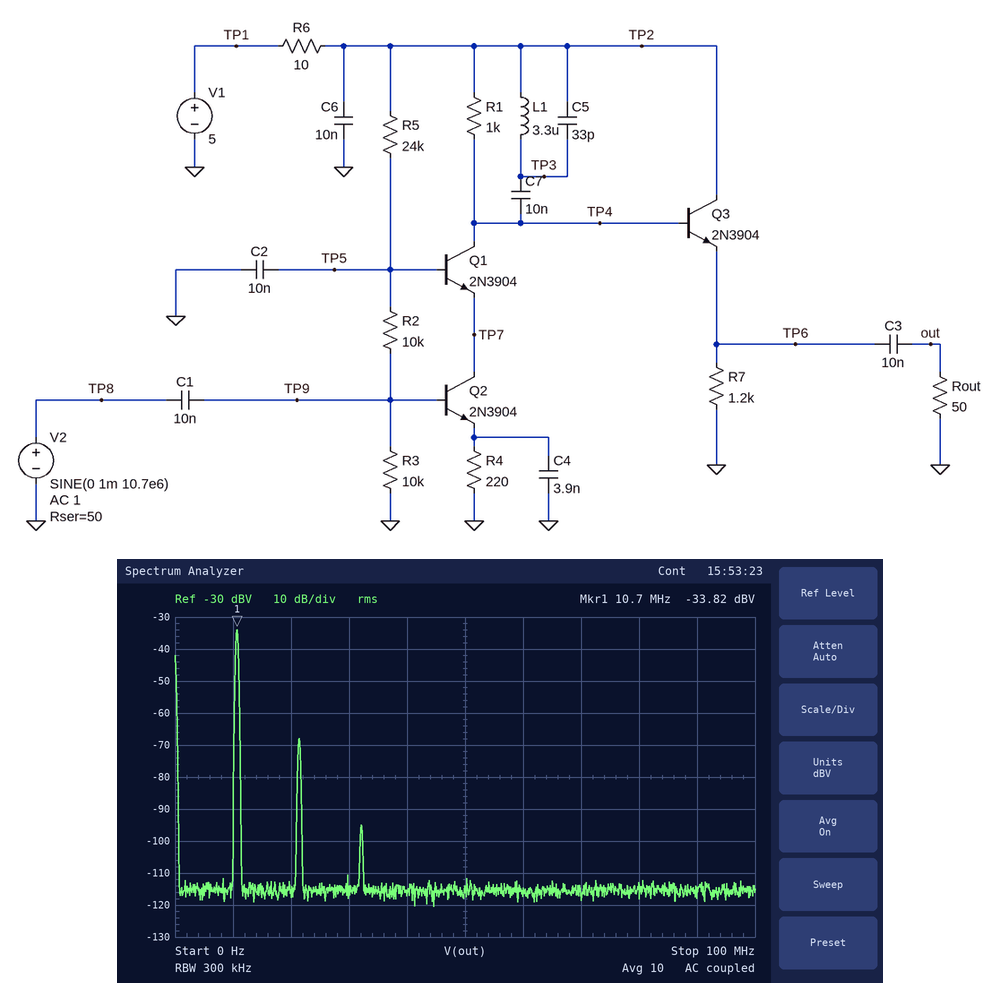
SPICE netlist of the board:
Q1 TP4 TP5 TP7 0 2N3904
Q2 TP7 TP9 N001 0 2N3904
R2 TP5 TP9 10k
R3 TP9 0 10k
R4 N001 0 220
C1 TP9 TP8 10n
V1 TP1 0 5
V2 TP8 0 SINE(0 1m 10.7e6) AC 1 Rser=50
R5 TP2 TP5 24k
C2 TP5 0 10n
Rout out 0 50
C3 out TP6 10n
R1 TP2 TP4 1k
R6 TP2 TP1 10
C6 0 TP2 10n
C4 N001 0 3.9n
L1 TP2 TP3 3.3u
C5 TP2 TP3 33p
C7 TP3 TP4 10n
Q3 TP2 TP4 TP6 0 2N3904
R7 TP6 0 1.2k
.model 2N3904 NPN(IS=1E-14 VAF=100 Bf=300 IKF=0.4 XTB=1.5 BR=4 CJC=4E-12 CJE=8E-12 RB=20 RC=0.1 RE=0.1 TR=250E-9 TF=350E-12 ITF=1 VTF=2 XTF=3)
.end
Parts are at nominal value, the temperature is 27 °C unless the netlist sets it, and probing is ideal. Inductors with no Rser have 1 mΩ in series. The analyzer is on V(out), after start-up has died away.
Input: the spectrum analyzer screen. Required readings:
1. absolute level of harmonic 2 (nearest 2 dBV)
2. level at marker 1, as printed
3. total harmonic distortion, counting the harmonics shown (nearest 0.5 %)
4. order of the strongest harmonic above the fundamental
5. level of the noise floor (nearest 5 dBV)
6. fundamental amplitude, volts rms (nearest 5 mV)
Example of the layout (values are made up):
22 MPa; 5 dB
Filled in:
-68 dBV; -33.82 dBV; 2.0 %; 2; -115 dBV; 20 mV
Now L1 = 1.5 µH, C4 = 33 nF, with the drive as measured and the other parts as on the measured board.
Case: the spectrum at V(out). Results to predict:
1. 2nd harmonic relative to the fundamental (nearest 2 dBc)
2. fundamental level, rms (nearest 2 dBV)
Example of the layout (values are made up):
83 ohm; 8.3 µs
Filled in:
-28 dBc; -46 dBV
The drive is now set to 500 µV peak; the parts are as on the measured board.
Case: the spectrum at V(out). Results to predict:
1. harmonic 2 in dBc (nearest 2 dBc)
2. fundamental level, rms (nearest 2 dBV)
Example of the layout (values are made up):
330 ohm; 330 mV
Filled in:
-40 dBc; -40 dBV
